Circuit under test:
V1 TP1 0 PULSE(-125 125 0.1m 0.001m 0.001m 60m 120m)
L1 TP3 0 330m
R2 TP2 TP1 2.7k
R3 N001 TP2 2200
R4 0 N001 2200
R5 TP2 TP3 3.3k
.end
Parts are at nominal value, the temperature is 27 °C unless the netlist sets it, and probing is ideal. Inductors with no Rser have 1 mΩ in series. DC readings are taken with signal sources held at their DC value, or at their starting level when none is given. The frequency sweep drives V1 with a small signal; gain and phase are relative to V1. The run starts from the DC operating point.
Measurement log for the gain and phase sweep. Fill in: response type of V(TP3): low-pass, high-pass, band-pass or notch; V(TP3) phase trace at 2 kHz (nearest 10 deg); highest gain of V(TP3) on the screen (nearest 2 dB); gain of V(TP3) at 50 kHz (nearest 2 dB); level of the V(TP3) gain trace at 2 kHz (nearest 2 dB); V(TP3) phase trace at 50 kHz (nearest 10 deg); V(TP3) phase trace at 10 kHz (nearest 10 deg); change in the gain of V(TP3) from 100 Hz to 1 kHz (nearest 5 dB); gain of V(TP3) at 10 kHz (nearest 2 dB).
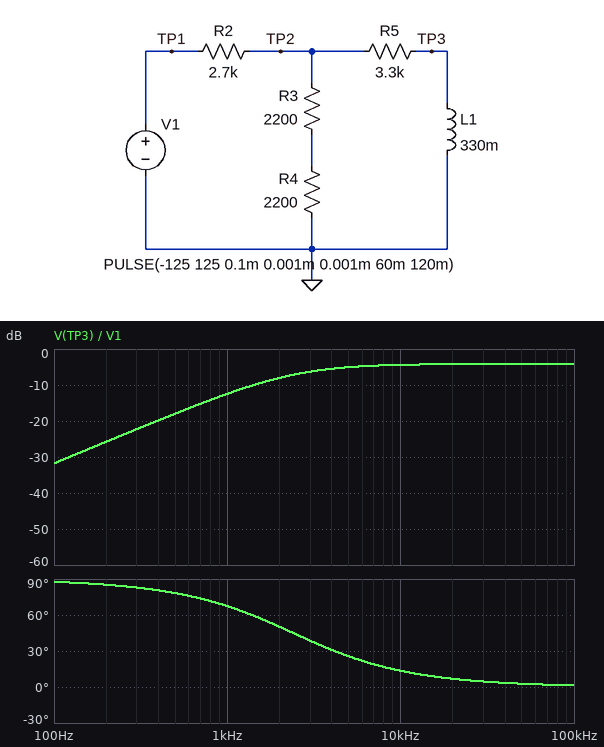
high-pass
50 deg
-4 dB
-4 dB
-8 dB
0 deg
10 deg
20 dB
-4 dB
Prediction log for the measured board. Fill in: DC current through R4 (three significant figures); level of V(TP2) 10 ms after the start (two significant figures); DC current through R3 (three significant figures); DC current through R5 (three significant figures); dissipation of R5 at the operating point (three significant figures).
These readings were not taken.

11.7 mA
51 V
11.7 mA
15.6 mA
801 mW
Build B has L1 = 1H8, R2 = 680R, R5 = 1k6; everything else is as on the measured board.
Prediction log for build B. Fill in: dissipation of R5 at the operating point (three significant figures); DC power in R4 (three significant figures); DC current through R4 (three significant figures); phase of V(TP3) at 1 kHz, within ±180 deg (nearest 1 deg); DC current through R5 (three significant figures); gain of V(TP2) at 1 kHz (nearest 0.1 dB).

3.91 W
712 mW
18.0 mA
11 deg
49.5 mA
-1.3 dB
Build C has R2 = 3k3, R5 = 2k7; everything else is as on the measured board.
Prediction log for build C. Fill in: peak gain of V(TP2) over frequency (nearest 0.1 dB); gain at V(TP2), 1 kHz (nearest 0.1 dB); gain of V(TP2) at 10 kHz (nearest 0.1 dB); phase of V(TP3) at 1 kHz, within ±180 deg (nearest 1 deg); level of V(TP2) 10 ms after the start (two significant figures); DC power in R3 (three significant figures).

-4.9 dB
-8.3 dB
-5.0 dB
66 deg
42 V
201 mW
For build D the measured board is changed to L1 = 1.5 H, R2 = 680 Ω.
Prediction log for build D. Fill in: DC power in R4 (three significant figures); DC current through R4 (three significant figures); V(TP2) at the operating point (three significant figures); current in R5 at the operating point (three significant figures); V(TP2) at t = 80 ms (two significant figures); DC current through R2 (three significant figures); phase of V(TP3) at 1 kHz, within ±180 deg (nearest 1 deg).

959 mW
20.9 mA
-91.9 V
27.8 mA
-92 V
48.7 mA
22 deg
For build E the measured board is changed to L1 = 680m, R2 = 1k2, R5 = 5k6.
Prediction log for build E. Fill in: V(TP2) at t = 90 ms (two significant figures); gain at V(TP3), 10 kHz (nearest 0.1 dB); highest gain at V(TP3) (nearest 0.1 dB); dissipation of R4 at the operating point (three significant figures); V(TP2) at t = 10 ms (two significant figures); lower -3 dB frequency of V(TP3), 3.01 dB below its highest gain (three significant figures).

-84 V
-2.2 dB
-2.1 dB
803 mW
84 V
1.53 kHz
